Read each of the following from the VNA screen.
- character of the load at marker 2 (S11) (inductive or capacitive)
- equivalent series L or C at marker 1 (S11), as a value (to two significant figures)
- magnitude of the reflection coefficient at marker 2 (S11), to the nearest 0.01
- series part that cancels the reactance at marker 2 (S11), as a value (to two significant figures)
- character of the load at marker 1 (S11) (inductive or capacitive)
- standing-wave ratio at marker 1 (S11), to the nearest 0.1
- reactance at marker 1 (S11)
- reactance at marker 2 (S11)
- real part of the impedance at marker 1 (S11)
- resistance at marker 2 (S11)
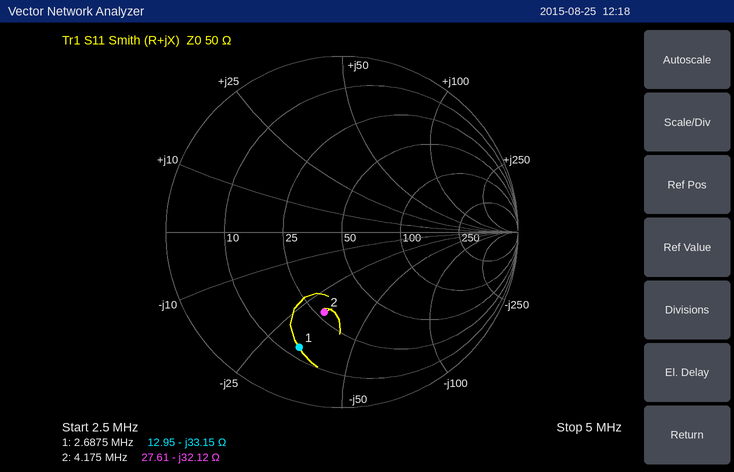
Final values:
capacitive
1.8 nF
0.47
1.2 µH
capacitive
5.6
-33.15 Ω
-32.12 Ω
12.95 Ω
27.61 Ω
